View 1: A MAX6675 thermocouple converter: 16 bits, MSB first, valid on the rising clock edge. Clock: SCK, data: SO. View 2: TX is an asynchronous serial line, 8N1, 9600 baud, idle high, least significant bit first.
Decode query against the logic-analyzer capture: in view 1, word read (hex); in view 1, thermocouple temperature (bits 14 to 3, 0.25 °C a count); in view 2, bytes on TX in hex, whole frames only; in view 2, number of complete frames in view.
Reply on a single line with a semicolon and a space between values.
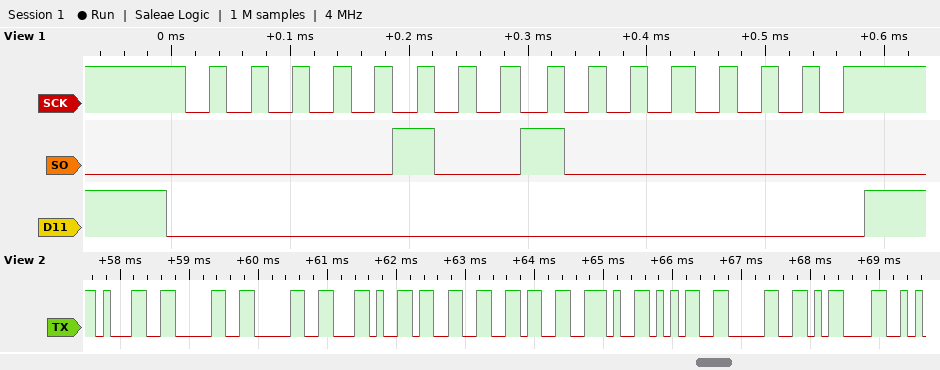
0x0480; 36.00 °C; 31 30 30 2C 33 36 2E 35 30 0D; 10
